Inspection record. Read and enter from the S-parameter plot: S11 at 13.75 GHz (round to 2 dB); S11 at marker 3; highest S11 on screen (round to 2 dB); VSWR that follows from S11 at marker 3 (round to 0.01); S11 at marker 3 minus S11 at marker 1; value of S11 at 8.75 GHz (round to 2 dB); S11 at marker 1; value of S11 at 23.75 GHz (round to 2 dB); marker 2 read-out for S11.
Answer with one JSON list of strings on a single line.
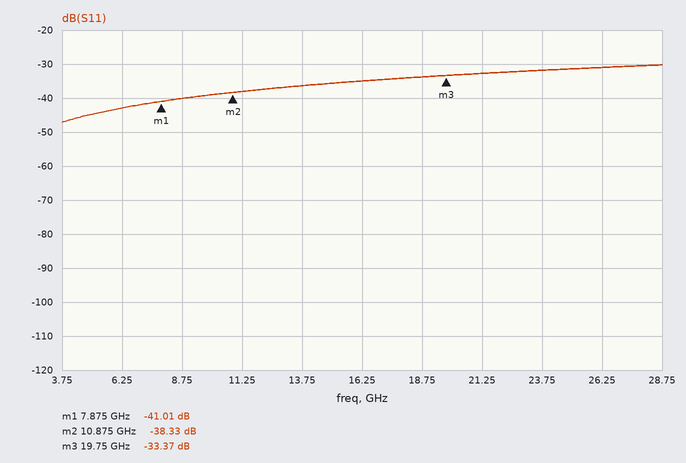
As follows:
["-36 dB", "-33.37 dB", "-30 dB", "1.04", "7.64 dB", "-40 dB", "-41.01 dB", "-32 dB", "-38.33 dB"]
